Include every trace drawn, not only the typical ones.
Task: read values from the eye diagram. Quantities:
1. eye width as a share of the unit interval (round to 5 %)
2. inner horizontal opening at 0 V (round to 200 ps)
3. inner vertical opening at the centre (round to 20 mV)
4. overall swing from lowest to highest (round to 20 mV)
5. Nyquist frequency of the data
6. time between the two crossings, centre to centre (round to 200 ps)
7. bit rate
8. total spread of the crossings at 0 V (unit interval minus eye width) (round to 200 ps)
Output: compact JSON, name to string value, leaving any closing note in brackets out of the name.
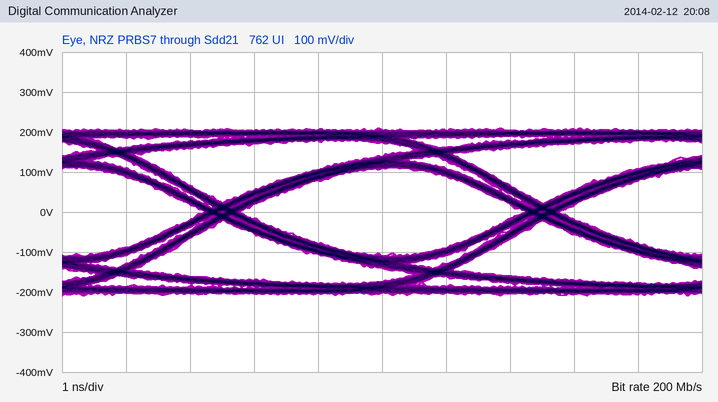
{"eye width as a share of the unit interval": "90 %", "inner horizontal opening at 0 V": "4.4 ns", "inner vertical opening at the centre": "220 mV", "overall swing from lowest to highest": "420 mV", "Nyquist frequency of the data": "100 MHz", "time between the two crossings, centre to centre": "5.0 ns", "bit rate": "200 Mb/s", "total spread of the crossings at 0 V (unit interval minus eye width)": "600 ps"}
